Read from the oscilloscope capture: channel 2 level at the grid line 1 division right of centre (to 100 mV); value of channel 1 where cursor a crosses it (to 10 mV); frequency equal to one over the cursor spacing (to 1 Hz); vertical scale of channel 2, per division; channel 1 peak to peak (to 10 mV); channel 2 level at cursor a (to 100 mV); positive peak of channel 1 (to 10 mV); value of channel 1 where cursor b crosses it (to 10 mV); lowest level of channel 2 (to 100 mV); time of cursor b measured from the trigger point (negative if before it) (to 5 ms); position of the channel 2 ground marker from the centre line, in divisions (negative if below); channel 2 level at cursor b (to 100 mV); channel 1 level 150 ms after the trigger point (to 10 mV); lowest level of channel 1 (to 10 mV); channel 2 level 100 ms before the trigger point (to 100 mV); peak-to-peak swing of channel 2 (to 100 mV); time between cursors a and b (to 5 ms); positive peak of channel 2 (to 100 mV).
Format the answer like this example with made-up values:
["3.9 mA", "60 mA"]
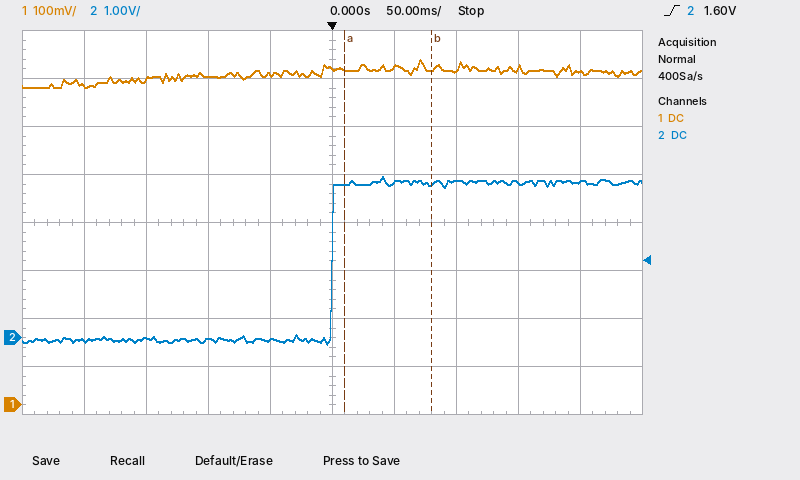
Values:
["3.2 V", "700 mV", "14 Hz", "1 V", "60 mV", "3.2 V", "720 mV", "700 mV", "-100 mV", "+80 ms", "-2.4 div", "3.2 V", "700 mV", "660 mV", "0.0 V", "3.5 V", "70 ms", "3.4 V"]
